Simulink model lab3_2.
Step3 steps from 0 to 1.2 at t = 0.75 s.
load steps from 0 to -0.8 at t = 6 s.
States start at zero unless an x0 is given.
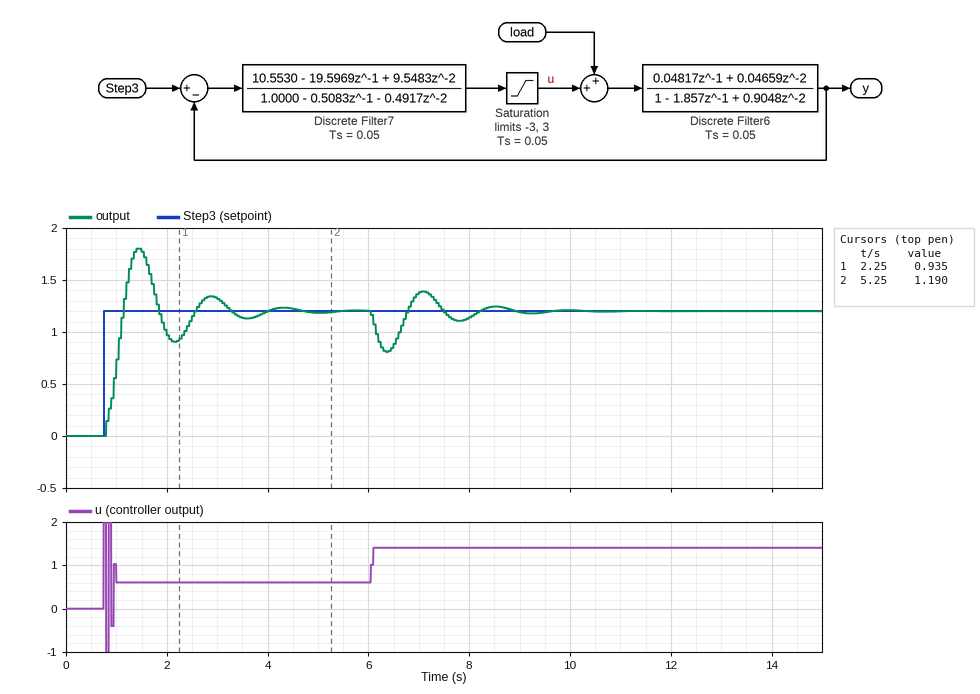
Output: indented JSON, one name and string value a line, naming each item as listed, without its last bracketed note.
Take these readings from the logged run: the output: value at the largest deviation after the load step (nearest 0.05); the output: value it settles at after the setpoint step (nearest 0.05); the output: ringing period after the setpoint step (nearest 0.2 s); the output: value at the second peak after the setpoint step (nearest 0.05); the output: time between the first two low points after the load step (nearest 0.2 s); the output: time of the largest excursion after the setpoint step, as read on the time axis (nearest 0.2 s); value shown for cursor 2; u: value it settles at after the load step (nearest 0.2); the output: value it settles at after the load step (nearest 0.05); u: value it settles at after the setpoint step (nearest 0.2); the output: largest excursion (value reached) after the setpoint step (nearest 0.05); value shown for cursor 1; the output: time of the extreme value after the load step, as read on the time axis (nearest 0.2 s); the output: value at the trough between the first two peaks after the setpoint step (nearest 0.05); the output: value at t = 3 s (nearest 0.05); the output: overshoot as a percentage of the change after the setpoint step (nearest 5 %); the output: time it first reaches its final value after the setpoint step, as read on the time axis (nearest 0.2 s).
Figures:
{
  "the output: value at the largest deviation after the load step": "0.80",
  "the output: value it settles at after the setpoint step": "1.20",
  "the output: ringing period after the setpoint step": "1.4 s",
  "the output: value at the second peak after the setpoint step": "1.35",
  "the output: time between the first two low points after the load step": "1.4 s",
  "the output: time of the largest excursion after the setpoint step, as read on the time axis": "1.4 s",
  "value shown for cursor 2": "1.190",
  "u: value it settles at after the load step": "1.4",
  "the output: value it settles at after the load step": "1.20",
  "u: value it settles at after the setpoint step": "0.6",
  "the output: largest excursion (value reached) after the setpoint step": "1.80",
  "value shown for cursor 1": "0.935",
  "the output: time of the extreme value after the load step, as read on the time axis": "6.4 s",
  "the output: value at the trough between the first two peaks after the setpoint step": "0.90",
  "the output: value at t = 3 s": "1.30",
  "the output: overshoot as a percentage of the change after the setpoint step": "50 %",
  "the output: time it first reaches its final value after the setpoint step, as read on the time axis": "1.2 s"
}
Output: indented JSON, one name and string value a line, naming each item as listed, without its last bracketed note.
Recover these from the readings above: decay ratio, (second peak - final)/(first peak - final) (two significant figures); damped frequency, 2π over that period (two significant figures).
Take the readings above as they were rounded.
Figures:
{
  "decay ratio, (second peak - final)/(first peak - final)": "0.25",
  "damped frequency, 2π over that period": "4.5 rad/s"
}
